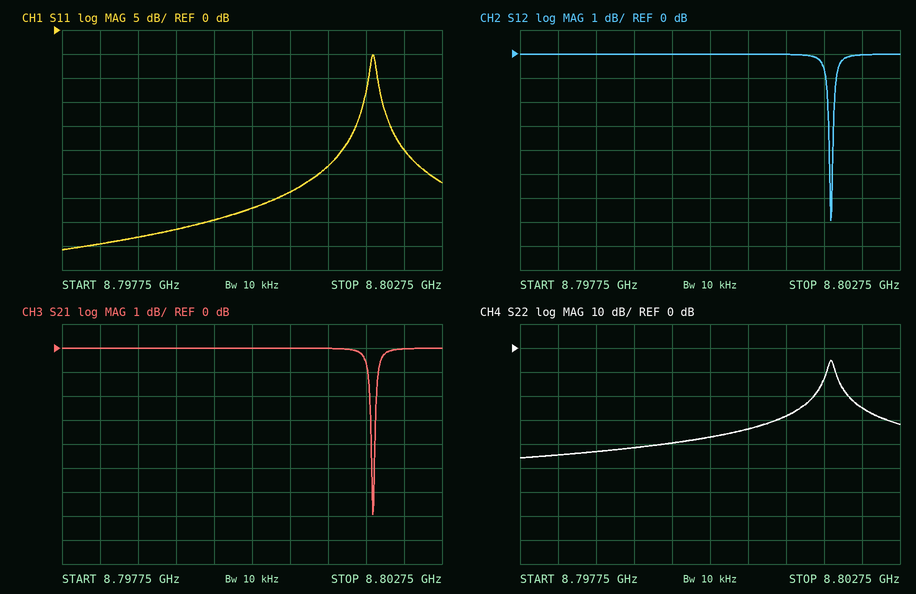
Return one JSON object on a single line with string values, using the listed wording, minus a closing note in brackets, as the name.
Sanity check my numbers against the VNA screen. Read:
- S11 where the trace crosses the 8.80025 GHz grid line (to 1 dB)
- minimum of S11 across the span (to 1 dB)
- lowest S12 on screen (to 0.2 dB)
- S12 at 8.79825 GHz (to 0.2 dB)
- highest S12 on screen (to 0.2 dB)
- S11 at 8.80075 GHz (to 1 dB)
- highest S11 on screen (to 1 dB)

{"S11 where the trace crosses the 8.80025 GHz grid line": "-37 dB", "minimum of S11 across the span": "-46 dB", "lowest S12 on screen": "-7.0 dB", "S12 at 8.79825 GHz": "0.0 dB", "highest S12 on screen": "0.0 dB", "S11 at 8.80075 GHz": "-34 dB", "highest S11 on screen": "-5 dB"}
